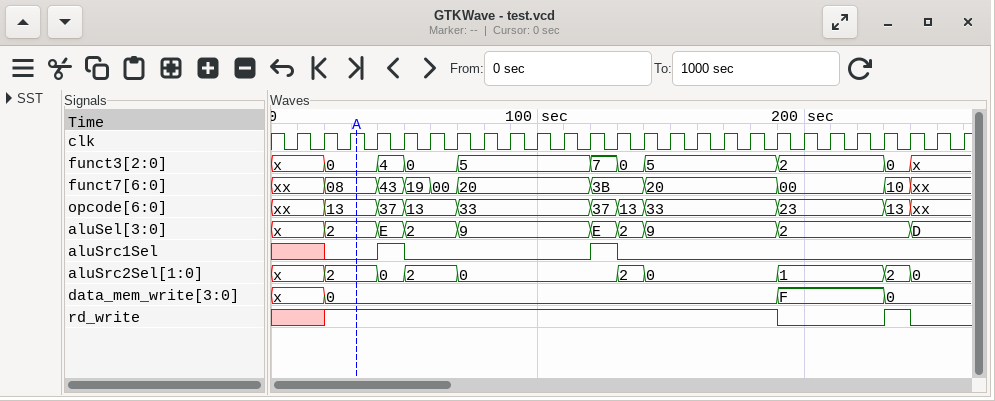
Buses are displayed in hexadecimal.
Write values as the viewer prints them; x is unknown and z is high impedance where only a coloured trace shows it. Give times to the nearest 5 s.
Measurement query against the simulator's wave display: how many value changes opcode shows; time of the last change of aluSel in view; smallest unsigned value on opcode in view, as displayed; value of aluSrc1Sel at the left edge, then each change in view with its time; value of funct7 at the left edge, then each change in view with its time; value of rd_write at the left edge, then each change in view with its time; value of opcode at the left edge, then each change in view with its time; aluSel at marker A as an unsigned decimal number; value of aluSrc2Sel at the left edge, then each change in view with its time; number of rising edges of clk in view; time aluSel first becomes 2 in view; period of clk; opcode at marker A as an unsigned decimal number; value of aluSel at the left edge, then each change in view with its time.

10
240 s
13
x, 0 at 20 s, 1 at 40 s, 0 at 50 s, 1 at 120 s, 0 at 130 s
xx, 08 at 20 s, 43 at 40 s, 19 at 50 s, 00 at 60 s, 20 at 70 s, 3B at 120 s, 20 at 140 s, 00 at 190 s, 10 at 230 s, xx at 240 s
x, 1 at 20 s, 0 at 190 s, 1 at 230 s, 0 at 240 s
xx, 13 at 20 s, 37 at 40 s, 13 at 50 s, 33 at 70 s, 37 at 120 s, 13 at 130 s, 33 at 140 s, 23 at 190 s, 13 at 230 s, xx at 240 s
2
x, 2 at 20 s, 0 at 40 s, 2 at 50 s, 0 at 70 s, 2 at 130 s, 0 at 140 s, 1 at 190 s, 2 at 230 s, 0 at 240 s
26
20 s
10 s
19
x, 2 at 20 s, E at 40 s, 2 at 50 s, 9 at 70 s, E at 120 s, 2 at 130 s, 9 at 140 s, 2 at 190 s, D at 240 s
